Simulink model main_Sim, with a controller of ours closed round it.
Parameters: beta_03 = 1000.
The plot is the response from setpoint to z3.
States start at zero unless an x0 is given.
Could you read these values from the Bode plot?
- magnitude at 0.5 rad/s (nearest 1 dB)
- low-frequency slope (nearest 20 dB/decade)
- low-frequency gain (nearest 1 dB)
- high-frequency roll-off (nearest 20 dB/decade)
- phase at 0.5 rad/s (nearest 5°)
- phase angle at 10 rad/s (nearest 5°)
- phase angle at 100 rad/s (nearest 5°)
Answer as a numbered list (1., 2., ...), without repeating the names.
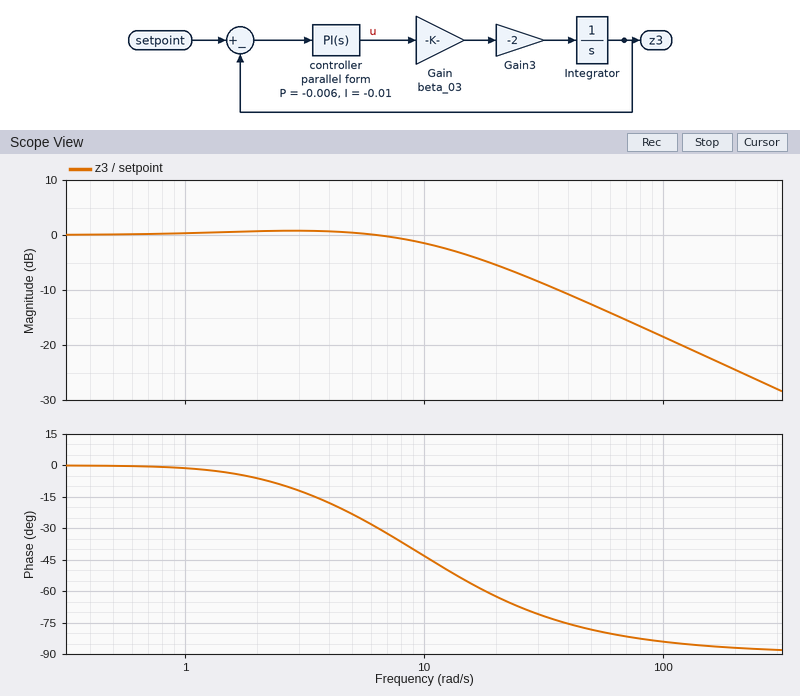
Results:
1. 0 dB
2. 0 dB/decade
3. 0 dB
4. -20 dB/decade
5. 0°
6. -45°
7. -85°
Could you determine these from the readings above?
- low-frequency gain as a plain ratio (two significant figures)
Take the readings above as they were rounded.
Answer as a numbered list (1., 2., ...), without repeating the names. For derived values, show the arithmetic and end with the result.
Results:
1. 10^(0 / 20) = 1.0
